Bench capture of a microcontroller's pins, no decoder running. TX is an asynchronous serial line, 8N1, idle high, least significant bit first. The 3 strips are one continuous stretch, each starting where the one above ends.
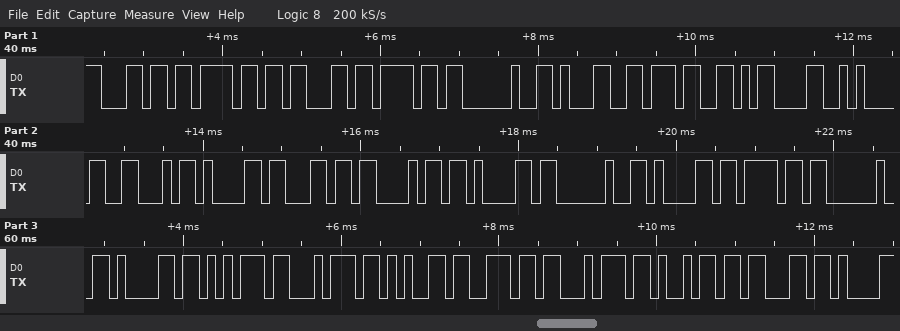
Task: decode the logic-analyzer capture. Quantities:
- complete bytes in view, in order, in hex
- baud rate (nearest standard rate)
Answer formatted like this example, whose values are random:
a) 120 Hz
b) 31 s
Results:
a) 6C 6F 63 6F 20 31 37 0D 0A 46 61 6C 68 61 20 61 6F 20 61 75 74 65 6E 74 69 63
b) 9600 baud
